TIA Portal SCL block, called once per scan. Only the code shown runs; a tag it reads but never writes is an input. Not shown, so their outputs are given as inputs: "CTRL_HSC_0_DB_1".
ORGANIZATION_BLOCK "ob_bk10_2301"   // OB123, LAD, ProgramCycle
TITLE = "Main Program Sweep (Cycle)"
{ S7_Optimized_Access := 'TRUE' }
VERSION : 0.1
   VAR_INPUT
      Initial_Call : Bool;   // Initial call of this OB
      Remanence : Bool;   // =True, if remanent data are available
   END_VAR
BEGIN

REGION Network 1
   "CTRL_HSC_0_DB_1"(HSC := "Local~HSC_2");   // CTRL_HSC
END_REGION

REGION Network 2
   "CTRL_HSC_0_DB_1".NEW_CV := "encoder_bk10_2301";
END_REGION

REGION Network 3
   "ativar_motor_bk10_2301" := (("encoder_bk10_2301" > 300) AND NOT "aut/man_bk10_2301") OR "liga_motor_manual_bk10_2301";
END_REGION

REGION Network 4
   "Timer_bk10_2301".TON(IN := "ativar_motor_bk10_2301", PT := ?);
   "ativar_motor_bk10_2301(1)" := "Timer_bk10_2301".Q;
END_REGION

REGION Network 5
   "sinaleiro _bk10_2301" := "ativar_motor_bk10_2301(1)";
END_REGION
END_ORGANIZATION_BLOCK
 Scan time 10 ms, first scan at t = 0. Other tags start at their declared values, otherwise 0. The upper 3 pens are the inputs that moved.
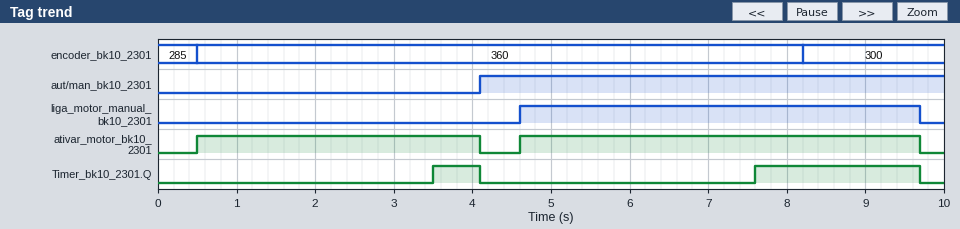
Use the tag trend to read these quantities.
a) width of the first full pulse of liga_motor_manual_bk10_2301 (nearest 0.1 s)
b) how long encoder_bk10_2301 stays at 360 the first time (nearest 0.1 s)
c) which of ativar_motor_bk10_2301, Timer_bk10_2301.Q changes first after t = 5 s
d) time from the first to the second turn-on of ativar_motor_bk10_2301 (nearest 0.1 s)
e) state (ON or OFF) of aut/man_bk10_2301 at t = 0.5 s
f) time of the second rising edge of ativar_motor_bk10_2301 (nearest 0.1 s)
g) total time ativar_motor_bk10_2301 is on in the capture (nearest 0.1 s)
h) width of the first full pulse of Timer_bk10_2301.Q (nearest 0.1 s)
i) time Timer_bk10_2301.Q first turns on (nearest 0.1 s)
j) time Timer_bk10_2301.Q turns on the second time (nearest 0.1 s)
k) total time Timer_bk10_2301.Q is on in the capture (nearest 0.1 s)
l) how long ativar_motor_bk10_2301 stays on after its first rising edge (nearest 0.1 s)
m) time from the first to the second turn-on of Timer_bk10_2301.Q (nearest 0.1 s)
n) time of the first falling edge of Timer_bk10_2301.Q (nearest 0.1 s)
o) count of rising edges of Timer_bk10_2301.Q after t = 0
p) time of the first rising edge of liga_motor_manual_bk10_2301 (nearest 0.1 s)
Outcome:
5.1 s
7.7 s
Timer_bk10_2301.Q
4.1 s
OFF
4.6 s
8.7 s
0.6 s
3.5 s
7.6 s
2.7 s
3.6 s
4.1 s
4.1 s
2
4.6 s
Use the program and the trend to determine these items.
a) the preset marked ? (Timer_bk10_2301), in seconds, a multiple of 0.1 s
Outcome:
3.0 s
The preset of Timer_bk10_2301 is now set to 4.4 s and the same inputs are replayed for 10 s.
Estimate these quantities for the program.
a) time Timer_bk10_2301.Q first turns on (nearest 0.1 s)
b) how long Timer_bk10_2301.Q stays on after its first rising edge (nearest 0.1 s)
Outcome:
9.0 s
0.7 s
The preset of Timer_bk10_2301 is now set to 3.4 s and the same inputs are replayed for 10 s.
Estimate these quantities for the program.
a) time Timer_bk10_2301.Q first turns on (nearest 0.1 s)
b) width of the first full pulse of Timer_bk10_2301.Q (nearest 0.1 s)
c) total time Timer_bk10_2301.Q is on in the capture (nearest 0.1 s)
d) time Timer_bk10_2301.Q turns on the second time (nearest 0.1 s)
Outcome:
3.9 s
0.2 s
1.9 s
8.0 s
